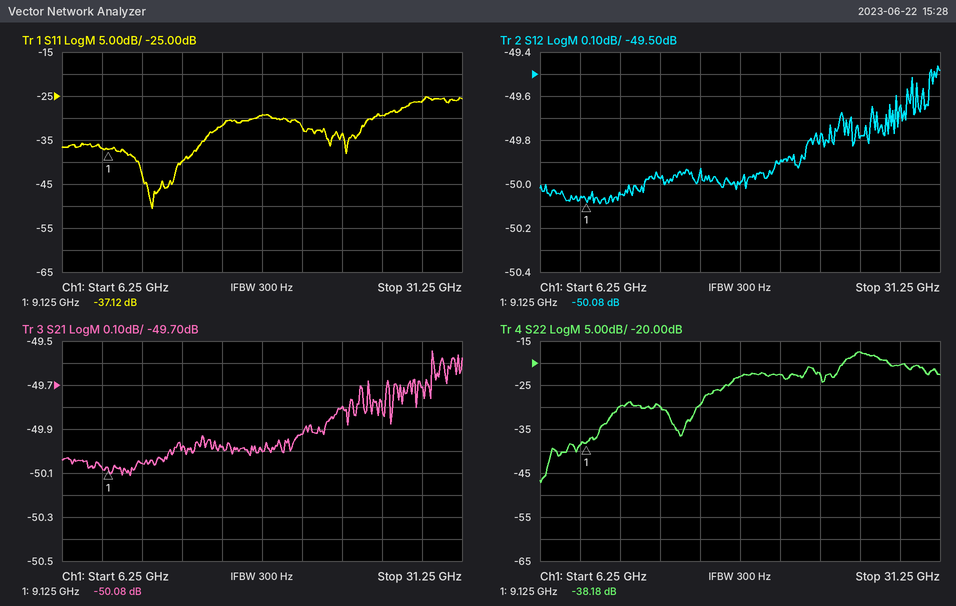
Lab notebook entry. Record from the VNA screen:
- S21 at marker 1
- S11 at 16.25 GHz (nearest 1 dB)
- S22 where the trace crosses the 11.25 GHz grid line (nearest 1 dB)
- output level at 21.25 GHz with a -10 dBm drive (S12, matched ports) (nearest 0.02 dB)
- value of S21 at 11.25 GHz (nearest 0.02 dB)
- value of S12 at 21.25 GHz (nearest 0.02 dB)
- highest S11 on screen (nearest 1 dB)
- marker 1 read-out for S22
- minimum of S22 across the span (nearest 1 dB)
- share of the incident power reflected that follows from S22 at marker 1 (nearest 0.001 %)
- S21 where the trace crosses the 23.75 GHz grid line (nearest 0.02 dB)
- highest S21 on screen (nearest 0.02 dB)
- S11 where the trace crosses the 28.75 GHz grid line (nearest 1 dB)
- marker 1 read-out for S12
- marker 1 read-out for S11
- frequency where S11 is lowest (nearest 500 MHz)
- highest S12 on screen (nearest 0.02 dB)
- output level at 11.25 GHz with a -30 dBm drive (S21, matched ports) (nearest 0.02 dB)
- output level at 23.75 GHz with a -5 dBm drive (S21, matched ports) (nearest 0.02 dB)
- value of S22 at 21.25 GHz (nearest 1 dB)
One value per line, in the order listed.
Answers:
-50.08 dB
-32 dB
-30 dB
-59.90 dBm
-50.06 dB
-49.90 dB
-25 dB
-38.18 dB
-47 dB
0.015 %
-49.80 dB
-49.54 dB
-26 dB
-50.08 dB
-37.12 dB
12.0 GHz
-49.46 dB
-80.06 dBm
-54.80 dBm
-23 dB
